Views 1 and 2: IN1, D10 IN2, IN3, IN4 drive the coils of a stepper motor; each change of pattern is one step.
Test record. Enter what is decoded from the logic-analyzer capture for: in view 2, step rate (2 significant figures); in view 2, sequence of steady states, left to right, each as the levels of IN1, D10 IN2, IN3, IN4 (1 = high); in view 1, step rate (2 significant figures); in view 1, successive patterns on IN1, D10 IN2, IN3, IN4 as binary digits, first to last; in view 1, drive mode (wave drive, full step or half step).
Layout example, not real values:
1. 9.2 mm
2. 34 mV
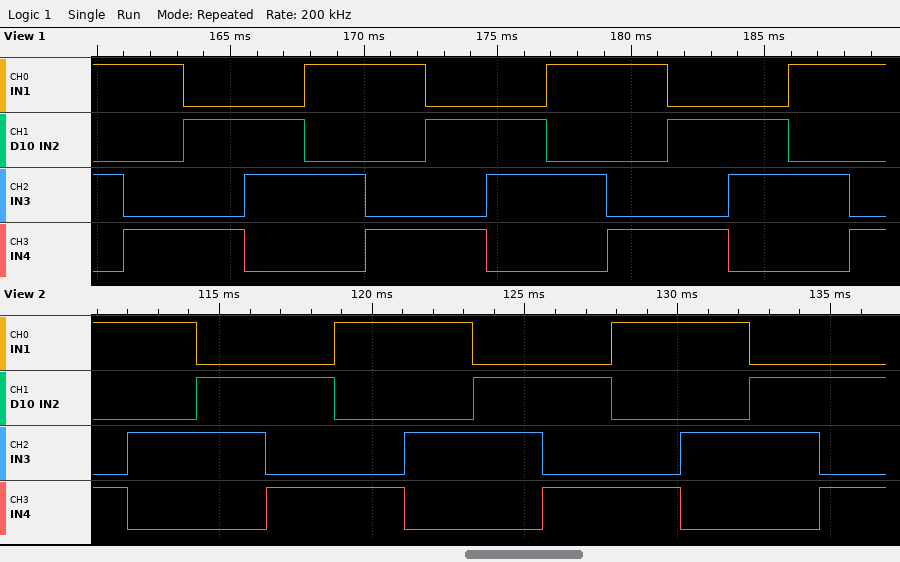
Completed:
1. 440 steps/s
2. 1001 1010 0110 0101 1001 1010 0110 0101 1001 1010 0110 0101
3. 440 steps/s
4. 1010 1001 0101 0110 1010 1001 0101 0110 1010 1001 0101 0110 1010 1001
5. full step
